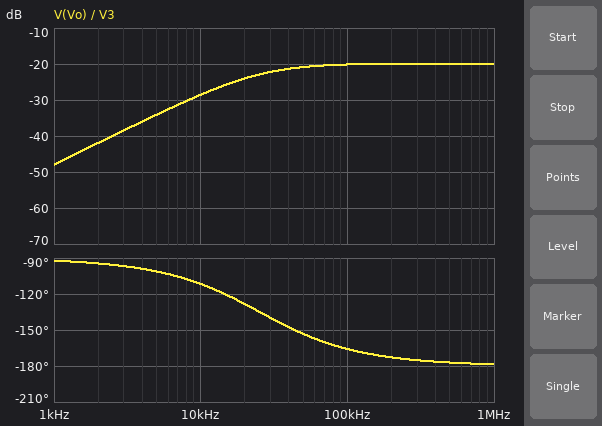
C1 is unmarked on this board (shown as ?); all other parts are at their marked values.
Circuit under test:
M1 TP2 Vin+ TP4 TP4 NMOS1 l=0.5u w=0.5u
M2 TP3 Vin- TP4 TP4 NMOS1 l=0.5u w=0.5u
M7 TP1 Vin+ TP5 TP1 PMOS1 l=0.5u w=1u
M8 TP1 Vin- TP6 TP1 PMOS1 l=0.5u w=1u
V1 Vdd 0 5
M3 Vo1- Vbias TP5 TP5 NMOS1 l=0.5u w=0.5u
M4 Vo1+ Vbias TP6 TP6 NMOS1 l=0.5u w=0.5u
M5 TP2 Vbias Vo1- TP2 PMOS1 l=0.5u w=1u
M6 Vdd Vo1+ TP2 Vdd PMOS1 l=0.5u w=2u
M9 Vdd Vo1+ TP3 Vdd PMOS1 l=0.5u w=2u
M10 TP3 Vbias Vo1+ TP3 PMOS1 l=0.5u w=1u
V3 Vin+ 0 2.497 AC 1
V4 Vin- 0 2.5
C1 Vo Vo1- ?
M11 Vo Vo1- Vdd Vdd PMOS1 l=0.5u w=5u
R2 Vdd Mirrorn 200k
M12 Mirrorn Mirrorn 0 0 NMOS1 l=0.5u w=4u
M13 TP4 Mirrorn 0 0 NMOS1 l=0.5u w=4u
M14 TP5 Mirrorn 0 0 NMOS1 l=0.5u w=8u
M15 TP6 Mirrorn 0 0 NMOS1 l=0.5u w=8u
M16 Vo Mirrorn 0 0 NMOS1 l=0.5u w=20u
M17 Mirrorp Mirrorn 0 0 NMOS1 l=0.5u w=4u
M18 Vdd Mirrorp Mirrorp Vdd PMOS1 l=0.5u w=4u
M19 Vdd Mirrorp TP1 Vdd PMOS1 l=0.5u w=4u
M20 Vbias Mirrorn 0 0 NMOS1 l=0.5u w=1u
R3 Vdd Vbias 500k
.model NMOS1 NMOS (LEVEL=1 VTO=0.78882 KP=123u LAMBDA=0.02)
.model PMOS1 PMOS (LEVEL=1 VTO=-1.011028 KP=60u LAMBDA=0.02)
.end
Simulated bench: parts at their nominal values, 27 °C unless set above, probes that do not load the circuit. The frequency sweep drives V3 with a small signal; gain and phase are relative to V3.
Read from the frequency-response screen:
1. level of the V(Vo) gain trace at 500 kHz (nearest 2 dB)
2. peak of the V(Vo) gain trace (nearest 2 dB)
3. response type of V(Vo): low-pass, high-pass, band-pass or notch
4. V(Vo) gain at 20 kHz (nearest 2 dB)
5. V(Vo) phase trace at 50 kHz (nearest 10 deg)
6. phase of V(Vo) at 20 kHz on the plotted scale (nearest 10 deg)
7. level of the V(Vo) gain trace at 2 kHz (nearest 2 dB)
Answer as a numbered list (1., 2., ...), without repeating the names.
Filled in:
1. -20 dB
2. -20 dB
3. high-pass
4. -24 dB
5. -150 deg
6. -130 deg
7. -42 dB
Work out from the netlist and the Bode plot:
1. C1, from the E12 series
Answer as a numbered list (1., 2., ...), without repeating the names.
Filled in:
1. 12 pF
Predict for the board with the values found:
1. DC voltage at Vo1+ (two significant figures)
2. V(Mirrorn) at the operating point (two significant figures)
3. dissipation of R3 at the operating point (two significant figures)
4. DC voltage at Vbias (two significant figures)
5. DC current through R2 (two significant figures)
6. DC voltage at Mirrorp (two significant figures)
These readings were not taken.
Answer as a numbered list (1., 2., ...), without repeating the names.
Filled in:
1. 3.4 V
2. 990 mV
3. 13 µW
4. 2.4 V
5. 20 µA
6. 3.7 V
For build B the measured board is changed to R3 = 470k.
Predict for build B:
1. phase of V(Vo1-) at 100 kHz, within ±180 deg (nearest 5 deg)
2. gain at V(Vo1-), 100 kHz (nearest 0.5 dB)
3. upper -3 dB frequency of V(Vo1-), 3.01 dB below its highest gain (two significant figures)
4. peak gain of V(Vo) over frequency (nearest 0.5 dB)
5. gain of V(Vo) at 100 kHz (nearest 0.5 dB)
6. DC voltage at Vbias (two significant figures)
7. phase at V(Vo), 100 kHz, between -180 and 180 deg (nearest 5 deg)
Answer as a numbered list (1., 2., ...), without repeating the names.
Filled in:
1. 125 deg
2. 20.5 dB
3. 65 kHz
4. -20.5 dB
5. -22.0 dB
6. 2.6 V
7. -145 deg
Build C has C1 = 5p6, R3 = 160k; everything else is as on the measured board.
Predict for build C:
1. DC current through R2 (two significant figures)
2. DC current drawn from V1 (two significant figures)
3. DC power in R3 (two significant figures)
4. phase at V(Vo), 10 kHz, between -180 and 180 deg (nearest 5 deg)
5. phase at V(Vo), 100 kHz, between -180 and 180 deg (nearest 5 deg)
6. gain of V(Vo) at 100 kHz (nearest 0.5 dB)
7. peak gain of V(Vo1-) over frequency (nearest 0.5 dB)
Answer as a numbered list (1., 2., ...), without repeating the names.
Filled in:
1. 20 µA
2. 200 µA
3. 4.5 µW
4. 0 deg
5. -10 deg
6. -61.0 dB
7. -22.0 dB
